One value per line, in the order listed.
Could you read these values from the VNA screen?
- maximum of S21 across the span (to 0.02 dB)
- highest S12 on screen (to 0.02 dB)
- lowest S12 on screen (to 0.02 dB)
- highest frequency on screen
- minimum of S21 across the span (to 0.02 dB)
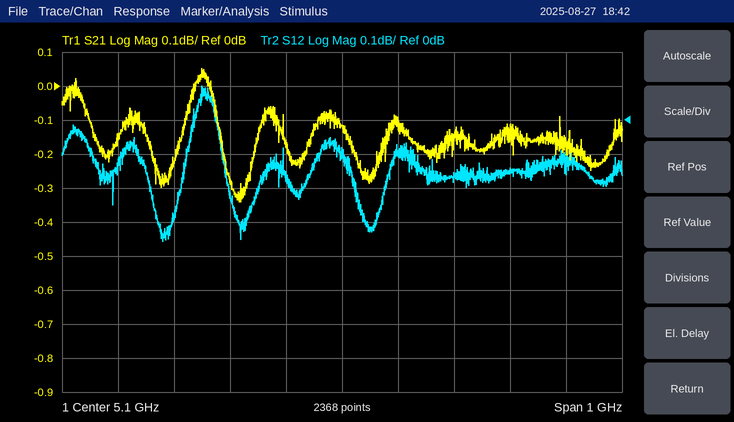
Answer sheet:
0.06 dB
0.10 dB
-0.36 dB
5.6 GHz
-0.34 dB
